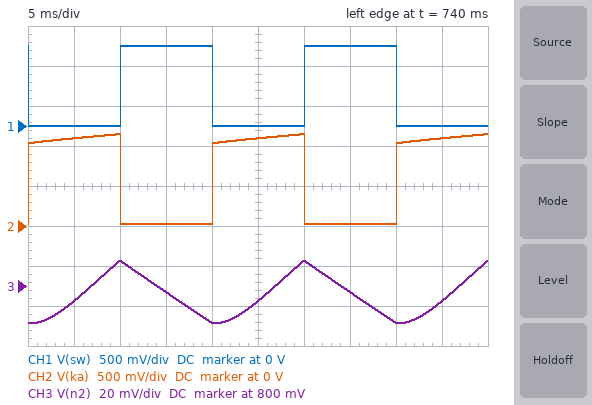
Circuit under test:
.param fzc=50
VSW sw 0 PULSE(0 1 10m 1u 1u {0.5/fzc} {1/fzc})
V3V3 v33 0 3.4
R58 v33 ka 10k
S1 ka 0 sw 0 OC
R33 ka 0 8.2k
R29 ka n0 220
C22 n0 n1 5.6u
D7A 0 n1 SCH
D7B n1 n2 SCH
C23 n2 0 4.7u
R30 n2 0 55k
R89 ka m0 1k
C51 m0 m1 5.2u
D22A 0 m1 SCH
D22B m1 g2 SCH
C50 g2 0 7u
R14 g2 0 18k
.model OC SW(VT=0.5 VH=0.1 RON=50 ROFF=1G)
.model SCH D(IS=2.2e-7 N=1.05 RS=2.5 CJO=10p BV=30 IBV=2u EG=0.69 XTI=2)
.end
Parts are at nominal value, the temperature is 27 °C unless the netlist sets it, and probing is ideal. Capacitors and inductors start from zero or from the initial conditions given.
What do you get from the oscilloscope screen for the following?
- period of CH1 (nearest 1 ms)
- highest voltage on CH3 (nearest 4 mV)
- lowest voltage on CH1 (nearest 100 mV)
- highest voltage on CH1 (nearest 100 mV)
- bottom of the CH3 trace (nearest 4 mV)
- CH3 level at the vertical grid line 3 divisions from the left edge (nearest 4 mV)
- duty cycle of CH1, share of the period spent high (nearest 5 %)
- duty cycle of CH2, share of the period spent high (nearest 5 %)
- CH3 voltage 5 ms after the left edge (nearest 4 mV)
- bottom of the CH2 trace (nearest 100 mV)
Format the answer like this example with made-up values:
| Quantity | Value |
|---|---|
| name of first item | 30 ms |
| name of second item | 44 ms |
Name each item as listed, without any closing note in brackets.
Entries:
| Quantity | Value |
|---|---|
| period of CH1 | 20 ms |
| highest voltage on CH3 | 812 mV |
| lowest voltage on CH1 | 0 V |
| highest voltage on CH1 | 1.0 V |
| bottom of the CH3 trace | 780 mV |
| CH3 level at the vertical grid line 3 divisions from the left edge | 796 mV |
| duty cycle of CH1, share of the period spent high | 50 % |
| duty cycle of CH2, share of the period spent high | 50 % |
| CH3 voltage 5 ms after the left edge | 792 mV |
| bottom of the CH2 trace | 0 V |
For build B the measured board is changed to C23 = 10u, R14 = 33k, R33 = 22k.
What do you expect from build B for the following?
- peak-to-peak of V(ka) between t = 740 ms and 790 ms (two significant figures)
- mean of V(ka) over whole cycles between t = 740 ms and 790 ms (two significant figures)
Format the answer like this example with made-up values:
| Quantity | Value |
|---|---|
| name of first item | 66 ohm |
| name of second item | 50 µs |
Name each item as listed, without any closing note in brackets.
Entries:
| Quantity | Value |
|---|---|
| peak-to-peak of V(ka) between t = 740 ms and 790 ms | 1.6 V |
| mean of V(ka) over whole cycles between t = 740 ms and 790 ms | 790 mV |
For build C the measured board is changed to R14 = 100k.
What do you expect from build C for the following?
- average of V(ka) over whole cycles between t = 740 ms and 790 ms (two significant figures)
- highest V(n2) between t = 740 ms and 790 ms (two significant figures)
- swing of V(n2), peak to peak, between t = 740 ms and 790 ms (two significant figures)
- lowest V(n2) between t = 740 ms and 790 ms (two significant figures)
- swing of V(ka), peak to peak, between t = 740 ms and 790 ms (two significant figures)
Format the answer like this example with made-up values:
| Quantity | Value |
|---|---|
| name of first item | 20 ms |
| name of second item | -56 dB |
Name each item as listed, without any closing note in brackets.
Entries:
| Quantity | Value |
|---|---|
| average of V(ka) over whole cycles between t = 740 ms and 790 ms | 650 mV |
| highest V(n2) between t = 740 ms and 790 ms | 980 mV |
| swing of V(n2), peak to peak, between t = 740 ms and 790 ms | 38 mV |
| lowest V(n2) between t = 740 ms and 790 ms | 940 mV |
| swing of V(ka), peak to peak, between t = 740 ms and 790 ms | 1.3 V |
